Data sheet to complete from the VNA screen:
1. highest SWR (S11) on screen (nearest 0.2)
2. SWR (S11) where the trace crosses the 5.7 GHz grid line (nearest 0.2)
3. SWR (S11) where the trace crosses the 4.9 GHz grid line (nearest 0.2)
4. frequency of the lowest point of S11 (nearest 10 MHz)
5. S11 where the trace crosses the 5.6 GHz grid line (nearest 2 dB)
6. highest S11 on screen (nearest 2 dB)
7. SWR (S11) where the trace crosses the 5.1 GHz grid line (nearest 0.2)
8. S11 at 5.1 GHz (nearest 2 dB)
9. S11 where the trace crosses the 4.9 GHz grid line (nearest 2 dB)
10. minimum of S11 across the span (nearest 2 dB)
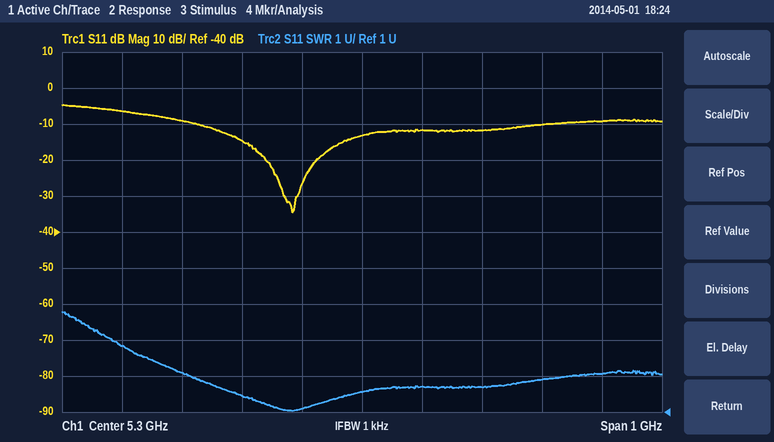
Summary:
3.8
2.0
2.8
5.18 GHz
-10 dB
-4 dB
1.4
-14 dB
-6 dB
-34 dB
